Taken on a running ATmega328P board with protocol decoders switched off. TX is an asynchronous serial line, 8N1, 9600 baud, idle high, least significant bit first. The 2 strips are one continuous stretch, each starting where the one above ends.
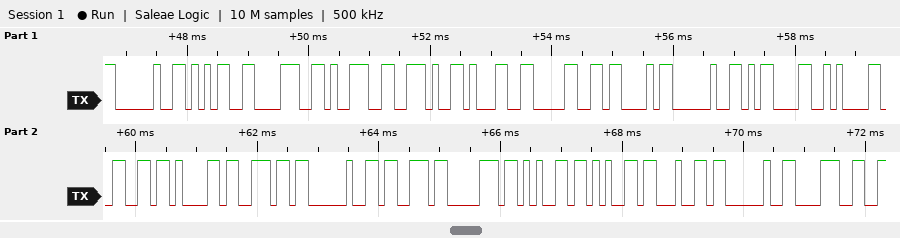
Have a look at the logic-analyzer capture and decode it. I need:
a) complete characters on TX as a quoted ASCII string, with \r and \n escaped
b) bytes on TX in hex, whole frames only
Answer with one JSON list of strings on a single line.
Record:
["\" 589.10C \\r\\nfan speed 8\"", "0x20 0x35 0x38 0x39 0x2E 0x31 0x30 0x43 0x20 0x0D 0x0A 0x66 0x61 0x6E 0x20 0x73 0x70 0x65 0x65 0x64 0x20 0x38"]
